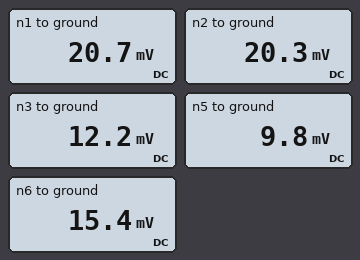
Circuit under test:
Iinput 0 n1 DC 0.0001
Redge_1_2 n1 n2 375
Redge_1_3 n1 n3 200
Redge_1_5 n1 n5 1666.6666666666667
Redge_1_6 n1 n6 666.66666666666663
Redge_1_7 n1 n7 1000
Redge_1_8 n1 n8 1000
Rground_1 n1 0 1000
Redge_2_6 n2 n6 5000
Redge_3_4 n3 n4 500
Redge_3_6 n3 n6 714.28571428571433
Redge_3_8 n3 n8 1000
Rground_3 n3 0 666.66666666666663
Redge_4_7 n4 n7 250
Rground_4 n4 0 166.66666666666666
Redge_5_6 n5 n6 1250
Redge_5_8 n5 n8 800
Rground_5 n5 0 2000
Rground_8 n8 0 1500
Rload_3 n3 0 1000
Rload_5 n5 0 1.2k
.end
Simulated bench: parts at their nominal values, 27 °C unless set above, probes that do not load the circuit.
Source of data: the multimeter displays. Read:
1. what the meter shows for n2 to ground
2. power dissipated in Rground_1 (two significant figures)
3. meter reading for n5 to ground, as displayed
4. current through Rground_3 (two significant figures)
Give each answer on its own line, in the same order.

20.3 mV
430 nW
9.8 mV
18 µA
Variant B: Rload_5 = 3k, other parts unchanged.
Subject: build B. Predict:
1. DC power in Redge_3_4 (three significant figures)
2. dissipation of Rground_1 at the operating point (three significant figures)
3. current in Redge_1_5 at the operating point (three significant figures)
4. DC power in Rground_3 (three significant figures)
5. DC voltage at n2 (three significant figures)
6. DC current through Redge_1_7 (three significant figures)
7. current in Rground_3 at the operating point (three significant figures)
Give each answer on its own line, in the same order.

124 nW
451 nW
5.63 µA
241 nW
20.9 mV
13.1 µA
19.0 µA
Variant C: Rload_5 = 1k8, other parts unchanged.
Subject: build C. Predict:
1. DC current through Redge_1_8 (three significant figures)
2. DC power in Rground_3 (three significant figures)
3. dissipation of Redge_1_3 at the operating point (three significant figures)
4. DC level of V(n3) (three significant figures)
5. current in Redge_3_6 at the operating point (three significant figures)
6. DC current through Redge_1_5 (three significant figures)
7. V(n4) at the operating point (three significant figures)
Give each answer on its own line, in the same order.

8.95 µA
233 nW
360 nW
12.5 mV
4.69 µA
6.06 µA
4.74 mV
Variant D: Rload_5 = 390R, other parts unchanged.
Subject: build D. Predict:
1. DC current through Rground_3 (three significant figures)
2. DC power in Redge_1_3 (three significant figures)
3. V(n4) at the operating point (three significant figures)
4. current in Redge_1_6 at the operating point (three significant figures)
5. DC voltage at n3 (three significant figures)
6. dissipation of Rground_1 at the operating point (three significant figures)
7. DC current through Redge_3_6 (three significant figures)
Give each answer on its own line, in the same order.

17.2 µA
333 nW
4.38 mV
8.56 µA
11.4 mV
384 nW
3.44 µA
